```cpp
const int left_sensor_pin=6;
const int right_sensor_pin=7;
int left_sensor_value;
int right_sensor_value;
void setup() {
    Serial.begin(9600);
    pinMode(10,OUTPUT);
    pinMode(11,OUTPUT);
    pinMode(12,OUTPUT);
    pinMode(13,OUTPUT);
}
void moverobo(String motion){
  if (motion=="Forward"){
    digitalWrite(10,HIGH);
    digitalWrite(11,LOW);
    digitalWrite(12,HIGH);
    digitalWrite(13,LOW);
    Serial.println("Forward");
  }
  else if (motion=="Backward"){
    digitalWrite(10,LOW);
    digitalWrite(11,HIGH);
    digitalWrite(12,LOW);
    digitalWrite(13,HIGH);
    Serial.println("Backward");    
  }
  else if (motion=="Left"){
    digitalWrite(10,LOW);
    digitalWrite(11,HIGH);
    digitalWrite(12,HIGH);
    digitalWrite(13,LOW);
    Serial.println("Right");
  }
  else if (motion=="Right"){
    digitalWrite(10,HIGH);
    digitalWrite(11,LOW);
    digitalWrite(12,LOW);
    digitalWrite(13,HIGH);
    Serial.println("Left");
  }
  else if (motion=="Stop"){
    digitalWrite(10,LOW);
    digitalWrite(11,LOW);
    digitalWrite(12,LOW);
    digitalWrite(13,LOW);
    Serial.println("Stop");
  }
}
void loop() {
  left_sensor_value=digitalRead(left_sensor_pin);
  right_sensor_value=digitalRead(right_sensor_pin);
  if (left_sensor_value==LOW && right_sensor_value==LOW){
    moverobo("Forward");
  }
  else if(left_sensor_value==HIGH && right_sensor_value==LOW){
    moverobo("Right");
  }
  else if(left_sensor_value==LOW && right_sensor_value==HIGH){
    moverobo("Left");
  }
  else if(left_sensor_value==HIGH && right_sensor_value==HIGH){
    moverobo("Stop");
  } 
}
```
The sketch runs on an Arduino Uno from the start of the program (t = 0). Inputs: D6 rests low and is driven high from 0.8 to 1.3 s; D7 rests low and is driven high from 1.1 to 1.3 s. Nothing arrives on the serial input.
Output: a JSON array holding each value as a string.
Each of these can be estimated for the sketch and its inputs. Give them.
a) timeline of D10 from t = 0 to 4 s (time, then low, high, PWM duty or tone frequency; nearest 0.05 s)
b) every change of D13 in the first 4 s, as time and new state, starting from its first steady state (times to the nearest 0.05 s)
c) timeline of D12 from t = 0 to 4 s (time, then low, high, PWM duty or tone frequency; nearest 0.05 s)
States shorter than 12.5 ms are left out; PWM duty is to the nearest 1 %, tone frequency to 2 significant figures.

["0 s high; 1.1 s low; 1.3 s high", "0 s low; 0.8 s high; 1.1 s low", "0 s high; 0.8 s low; 1.3 s high"]
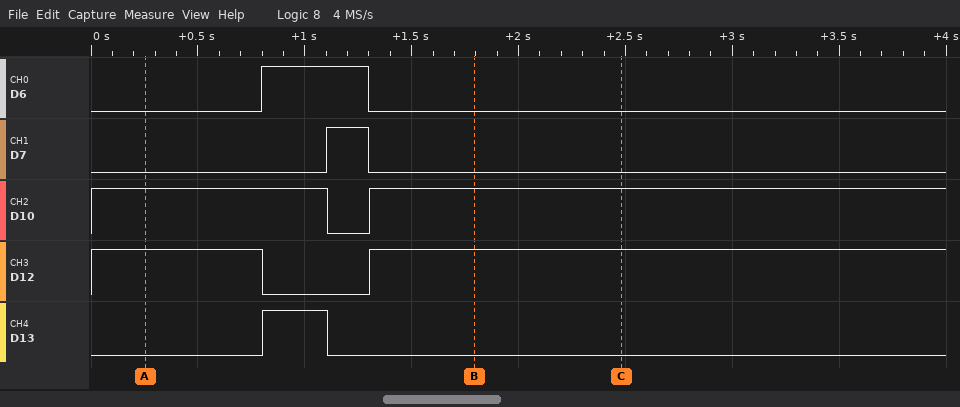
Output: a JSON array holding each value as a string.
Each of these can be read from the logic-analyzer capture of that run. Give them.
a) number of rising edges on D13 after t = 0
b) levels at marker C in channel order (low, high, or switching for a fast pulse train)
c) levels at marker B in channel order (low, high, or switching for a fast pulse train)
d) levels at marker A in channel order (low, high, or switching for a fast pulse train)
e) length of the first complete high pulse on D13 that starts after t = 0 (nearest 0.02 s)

["1", "D6 low, D7 low, D10 high, D12 high, D13 low", "D6 low, D7 low, D10 high, D12 high, D13 low", "D6 low, D7 low, D10 high, D12 high, D13 low", "0.30 s"]
